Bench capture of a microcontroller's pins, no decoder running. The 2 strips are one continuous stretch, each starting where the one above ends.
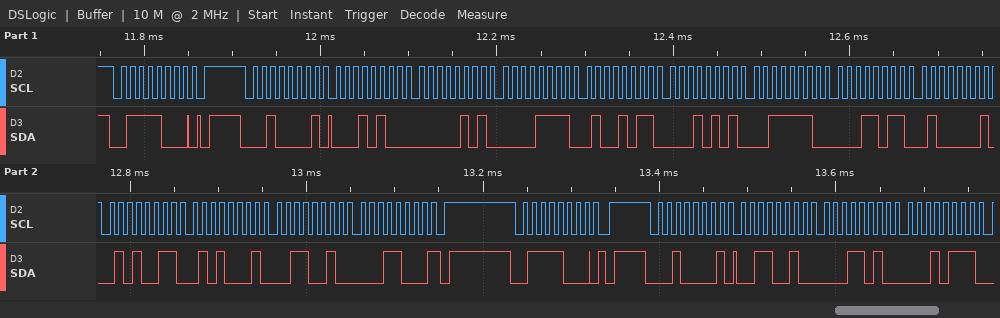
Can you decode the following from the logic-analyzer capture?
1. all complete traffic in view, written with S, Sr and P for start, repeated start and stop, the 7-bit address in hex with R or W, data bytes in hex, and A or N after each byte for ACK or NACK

S 3CW A P S 10R A 14 A 05 A 0F A 4B A 15 A 3E A 1B A 41 A 53 A 51 A 32 A 18 N P S 3CW A P S 10R A 32 A 1A A 17 A
